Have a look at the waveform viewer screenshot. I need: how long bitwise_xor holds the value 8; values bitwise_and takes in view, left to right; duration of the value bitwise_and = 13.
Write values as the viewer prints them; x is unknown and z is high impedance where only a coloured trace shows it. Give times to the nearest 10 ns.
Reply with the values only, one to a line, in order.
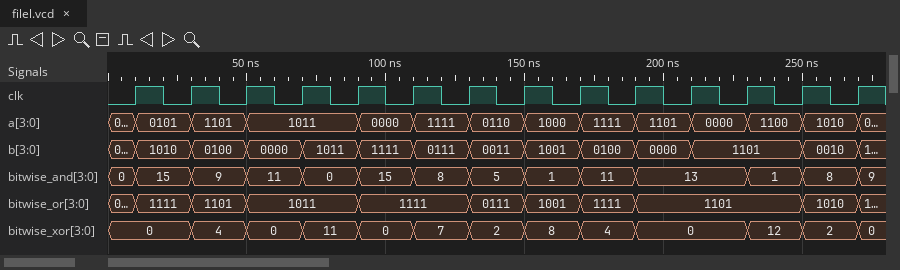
20 ns
0, 15, 9, 11, 0, 15, 8, 5, 1, 11, 13, 1, 8, 9
40 ns
